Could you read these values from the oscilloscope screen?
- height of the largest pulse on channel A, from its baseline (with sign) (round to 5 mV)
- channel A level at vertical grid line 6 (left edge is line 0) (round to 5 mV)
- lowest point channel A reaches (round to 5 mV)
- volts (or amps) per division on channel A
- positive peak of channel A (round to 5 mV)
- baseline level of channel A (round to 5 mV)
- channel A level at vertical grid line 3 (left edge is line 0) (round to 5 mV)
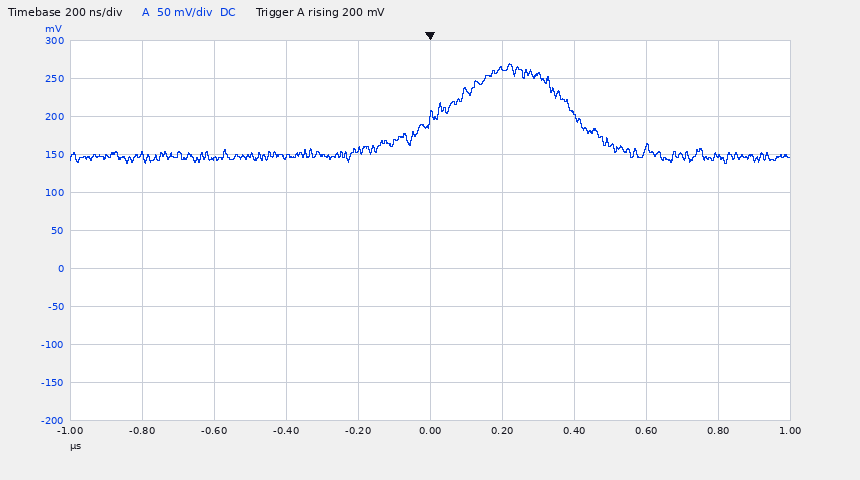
+120 mV
265 mV
140 mV
50 mV
270 mV
150 mV
145 mV
